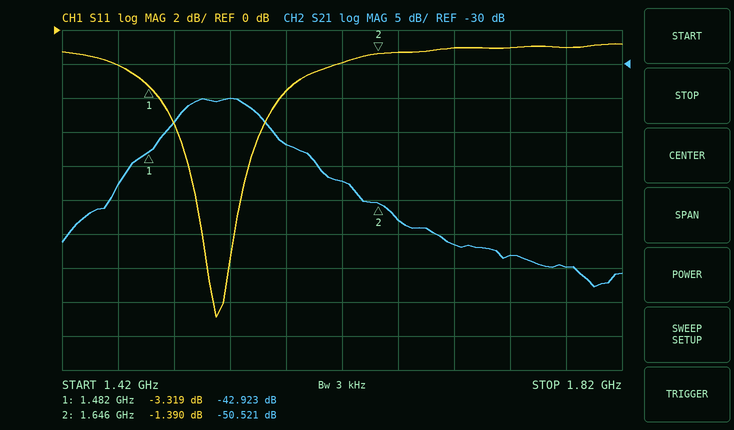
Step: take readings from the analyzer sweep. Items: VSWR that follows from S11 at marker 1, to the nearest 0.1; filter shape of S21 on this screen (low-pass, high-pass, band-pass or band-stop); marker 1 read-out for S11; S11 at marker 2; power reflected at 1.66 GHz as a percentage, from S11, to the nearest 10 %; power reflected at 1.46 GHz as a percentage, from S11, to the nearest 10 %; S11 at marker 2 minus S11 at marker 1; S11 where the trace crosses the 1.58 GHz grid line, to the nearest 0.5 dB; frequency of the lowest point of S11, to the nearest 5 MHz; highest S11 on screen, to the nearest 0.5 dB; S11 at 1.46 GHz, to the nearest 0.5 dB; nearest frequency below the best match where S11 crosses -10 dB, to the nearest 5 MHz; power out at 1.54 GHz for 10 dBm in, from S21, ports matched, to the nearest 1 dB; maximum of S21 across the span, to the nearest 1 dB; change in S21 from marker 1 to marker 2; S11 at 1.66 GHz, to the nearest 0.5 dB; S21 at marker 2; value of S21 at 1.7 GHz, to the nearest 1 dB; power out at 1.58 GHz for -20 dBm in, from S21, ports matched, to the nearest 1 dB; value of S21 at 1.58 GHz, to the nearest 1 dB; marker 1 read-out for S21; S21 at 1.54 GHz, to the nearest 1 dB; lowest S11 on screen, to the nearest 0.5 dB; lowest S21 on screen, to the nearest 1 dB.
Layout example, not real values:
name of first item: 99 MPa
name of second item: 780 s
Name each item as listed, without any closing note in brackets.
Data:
VSWR that follows from S11 at marker 1, to the nearest 0.1: 5.3
filter shape of S21 on this screen: band-pass
marker 1 read-out for S11: -3.319 dB
S11 at marker 2: -1.390 dB
power reflected at 1.66 GHz as a percentage, from S11, to the nearest 10 %: 70 %
power reflected at 1.46 GHz as a percentage, from S11, to the nearest 10 %: 60 %
S11 at marker 2 minus S11 at marker 1: 1.929 dB
S11 where the trace crosses the 1.58 GHz grid line, to the nearest 0.5 dB: -3.5 dB
frequency of the lowest point of S11, to the nearest 5 MHz: 1.530 GHz
highest S11 on screen, to the nearest 0.5 dB: -1.0 dB
S11 at 1.46 GHz, to the nearest 0.5 dB: -2.0 dB
nearest frequency below the best match where S11 crosses -10 dB, to the nearest 5 MHz: 1.515 GHz
power out at 1.54 GHz for 10 dBm in, from S21, ports matched, to the nearest 1 dB: -25 dBm
maximum of S21 across the span, to the nearest 1 dB: -35 dB
change in S21 from marker 1 to marker 2: -7.598 dB
S11 at 1.66 GHz, to the nearest 0.5 dB: -1.5 dB
S21 at marker 2: -50.521 dB
value of S21 at 1.7 GHz, to the nearest 1 dB: -57 dB
power out at 1.58 GHz for -20 dBm in, from S21, ports matched, to the nearest 1 dB: -62 dBm
value of S21 at 1.58 GHz, to the nearest 1 dB: -42 dB
marker 1 read-out for S21: -42.923 dB
S21 at 1.54 GHz, to the nearest 1 dB: -35 dB
lowest S11 on screen, to the nearest 0.5 dB: -17.0 dB
lowest S21 on screen, to the nearest 1 dB: -63 dB
